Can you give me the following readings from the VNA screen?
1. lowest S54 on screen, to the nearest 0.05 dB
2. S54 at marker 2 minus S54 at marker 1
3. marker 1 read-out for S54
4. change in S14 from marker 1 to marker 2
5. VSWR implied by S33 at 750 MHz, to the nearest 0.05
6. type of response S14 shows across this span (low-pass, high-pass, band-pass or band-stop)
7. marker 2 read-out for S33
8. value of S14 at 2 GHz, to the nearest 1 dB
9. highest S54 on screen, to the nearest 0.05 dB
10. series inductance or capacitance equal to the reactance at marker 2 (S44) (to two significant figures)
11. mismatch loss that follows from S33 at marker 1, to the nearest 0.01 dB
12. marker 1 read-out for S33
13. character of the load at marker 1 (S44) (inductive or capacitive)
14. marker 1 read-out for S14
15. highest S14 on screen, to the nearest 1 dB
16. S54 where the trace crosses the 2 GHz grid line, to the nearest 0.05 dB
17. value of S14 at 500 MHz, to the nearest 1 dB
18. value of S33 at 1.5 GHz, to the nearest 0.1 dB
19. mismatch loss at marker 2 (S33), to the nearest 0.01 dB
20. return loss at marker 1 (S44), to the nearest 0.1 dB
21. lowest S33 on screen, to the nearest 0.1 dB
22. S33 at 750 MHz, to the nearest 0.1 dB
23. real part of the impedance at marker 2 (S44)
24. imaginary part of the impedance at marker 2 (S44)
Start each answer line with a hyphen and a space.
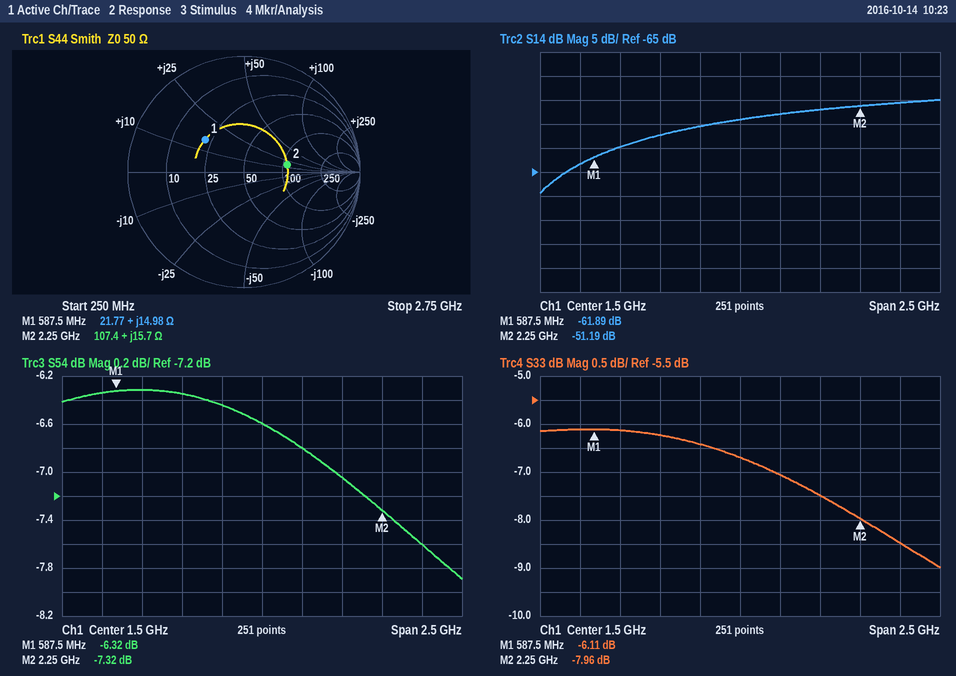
- -7.90 dB
- -1.00 dB
- -6.32 dB
- 10.70 dB
- 2.95
- high-pass
- -7.96 dB
- -52 dB
- -6.30 dB
- 1.1 nH
- 1.22 dB
- -6.11 dB
- inductive
- -61.89 dB
- -50 dB
- -7.05 dB
- -63 dB
- -6.7 dB
- 0.76 dB
- 7.2 dB
- -9.0 dB
- -6.1 dB
- 107.4 Ω
- +15.7 Ω
